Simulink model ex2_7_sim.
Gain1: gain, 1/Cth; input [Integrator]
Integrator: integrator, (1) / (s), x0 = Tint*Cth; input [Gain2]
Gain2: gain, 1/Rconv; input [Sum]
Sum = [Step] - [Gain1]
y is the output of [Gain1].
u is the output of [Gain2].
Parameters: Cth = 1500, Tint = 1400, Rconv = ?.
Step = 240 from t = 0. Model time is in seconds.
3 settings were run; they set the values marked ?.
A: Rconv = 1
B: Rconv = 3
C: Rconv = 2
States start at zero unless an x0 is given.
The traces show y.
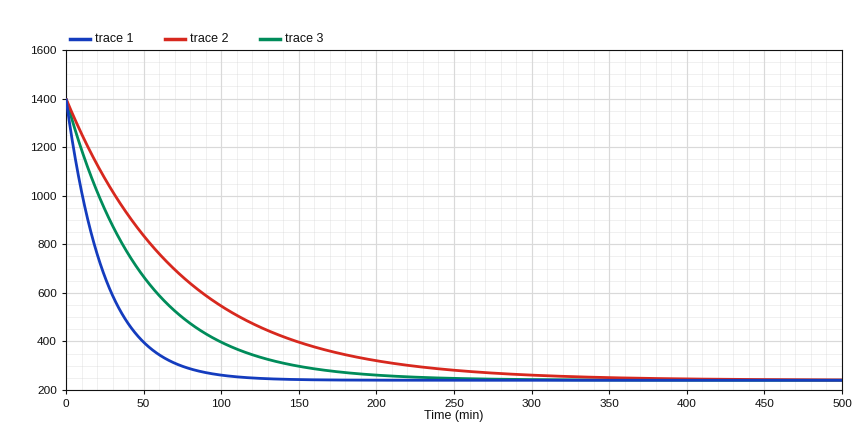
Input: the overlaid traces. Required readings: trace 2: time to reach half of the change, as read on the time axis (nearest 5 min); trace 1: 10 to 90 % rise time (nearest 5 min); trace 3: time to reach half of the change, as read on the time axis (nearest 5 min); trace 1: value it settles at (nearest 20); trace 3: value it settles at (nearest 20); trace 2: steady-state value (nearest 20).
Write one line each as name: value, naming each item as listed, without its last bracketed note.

trace 2: time to reach half of the change, as read on the time axis: 50 min
trace 1: 10 to 90 % rise time: 55 min
trace 3: time to reach half of the change, as read on the time axis: 35 min
trace 1: value it settles at: 240
trace 3: value it settles at: 240
trace 2: steady-state value: 240
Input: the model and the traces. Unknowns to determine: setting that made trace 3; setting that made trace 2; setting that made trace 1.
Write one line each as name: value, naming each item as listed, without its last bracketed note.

setting that made trace 3: C
setting that made trace 2: B
setting that made trace 1: A
